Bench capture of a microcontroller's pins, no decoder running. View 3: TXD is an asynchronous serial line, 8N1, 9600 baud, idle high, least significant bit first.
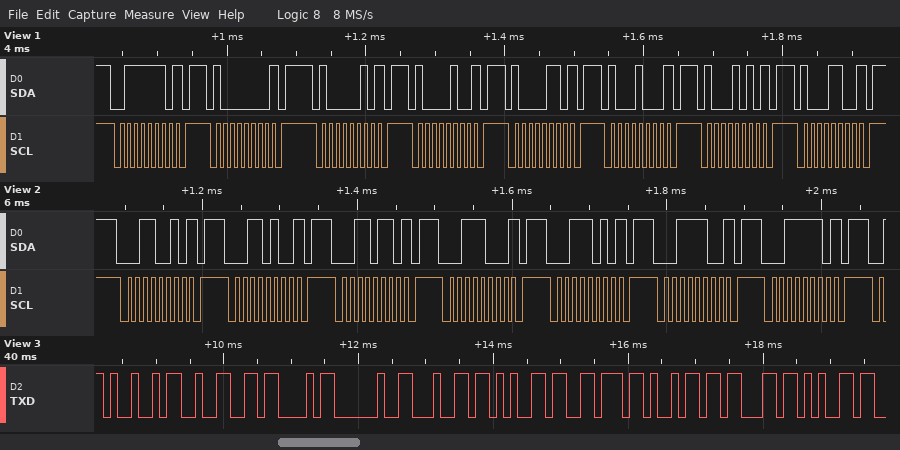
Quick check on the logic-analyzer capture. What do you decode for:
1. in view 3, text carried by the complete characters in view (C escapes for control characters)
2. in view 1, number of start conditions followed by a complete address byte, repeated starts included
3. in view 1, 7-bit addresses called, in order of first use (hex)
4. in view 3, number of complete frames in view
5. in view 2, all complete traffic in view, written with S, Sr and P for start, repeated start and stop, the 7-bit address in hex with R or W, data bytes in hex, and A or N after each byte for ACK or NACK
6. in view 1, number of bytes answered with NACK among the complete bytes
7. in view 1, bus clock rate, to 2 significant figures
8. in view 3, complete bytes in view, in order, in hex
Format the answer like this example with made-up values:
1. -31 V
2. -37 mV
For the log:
1. "I2C device"
2. 8
3. 0x3F 0x40 0x41 0x42 0x43 0x44 0x45 0x46
4. 10
5. S 19W N P S 1AW N P S 1BW N P S 1CW N P S 1DW N P S 1EW N P S 1FW N P
6. 8
7. 100 kHz
8. 49 32 43 20 64 65 76 69 63 65
